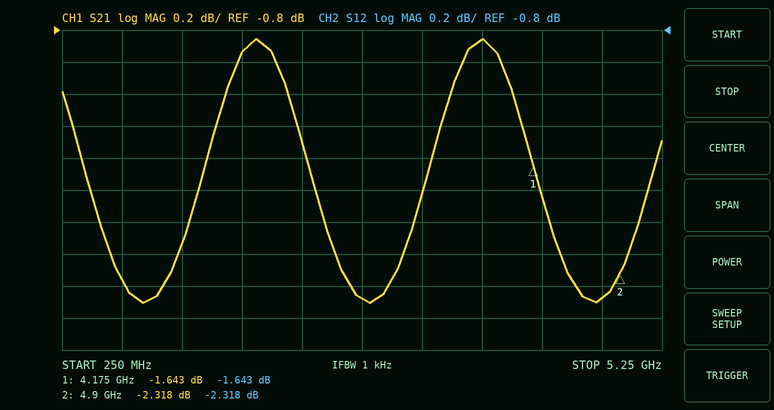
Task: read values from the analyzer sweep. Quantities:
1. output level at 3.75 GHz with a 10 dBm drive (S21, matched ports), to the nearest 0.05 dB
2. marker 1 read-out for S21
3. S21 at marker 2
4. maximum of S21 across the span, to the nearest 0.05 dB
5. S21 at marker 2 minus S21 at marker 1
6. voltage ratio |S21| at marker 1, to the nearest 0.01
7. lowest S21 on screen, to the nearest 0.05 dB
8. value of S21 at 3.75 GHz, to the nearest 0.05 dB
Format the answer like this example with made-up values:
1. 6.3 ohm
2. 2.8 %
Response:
1. 9.15 dBm
2. -1.643 dB
3. -2.318 dB
4. -0.85 dB
5. -0.675 dB
6. 0.83
7. -2.50 dB
8. -0.85 dB
